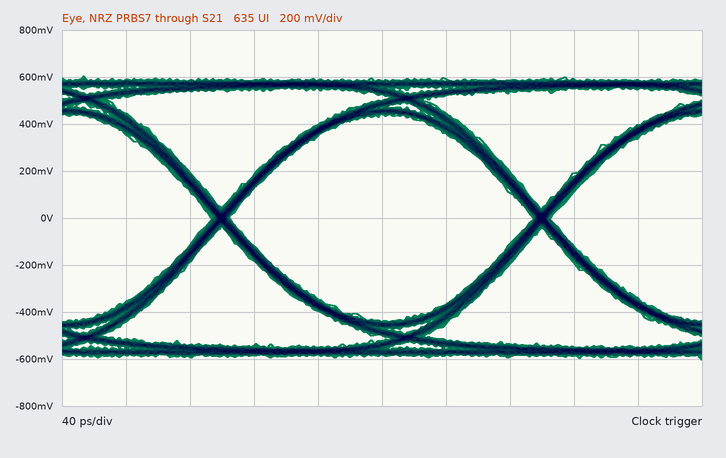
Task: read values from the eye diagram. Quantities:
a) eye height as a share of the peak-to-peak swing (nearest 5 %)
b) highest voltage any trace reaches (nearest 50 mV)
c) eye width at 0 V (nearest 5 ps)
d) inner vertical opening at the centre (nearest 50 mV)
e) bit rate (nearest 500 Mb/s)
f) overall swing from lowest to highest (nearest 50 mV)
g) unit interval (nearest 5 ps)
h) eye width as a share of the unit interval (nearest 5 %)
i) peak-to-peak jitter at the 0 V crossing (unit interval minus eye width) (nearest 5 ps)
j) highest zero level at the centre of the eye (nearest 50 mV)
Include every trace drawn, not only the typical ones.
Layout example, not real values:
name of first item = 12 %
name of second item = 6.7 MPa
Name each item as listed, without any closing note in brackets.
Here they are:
eye height as a share of the peak-to-peak swing = 75 %
highest voltage any trace reaches = 600 mV
eye width at 0 V = 190 ps
inner vertical opening at the centre = 900 mV
bit rate = 5.0 Gb/s
overall swing from lowest to highest = 1.20 V
unit interval = 200 ps
eye width as a share of the unit interval = 95 %
peak-to-peak jitter at the 0 V crossing (unit interval minus eye width) = 10 ps
highest zero level at the centre of the eye = -450 mV
